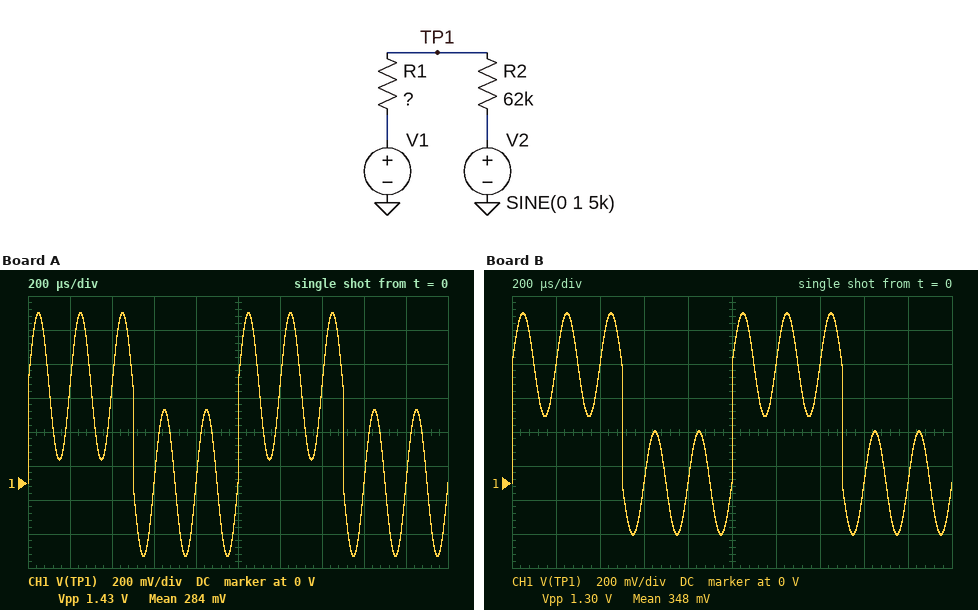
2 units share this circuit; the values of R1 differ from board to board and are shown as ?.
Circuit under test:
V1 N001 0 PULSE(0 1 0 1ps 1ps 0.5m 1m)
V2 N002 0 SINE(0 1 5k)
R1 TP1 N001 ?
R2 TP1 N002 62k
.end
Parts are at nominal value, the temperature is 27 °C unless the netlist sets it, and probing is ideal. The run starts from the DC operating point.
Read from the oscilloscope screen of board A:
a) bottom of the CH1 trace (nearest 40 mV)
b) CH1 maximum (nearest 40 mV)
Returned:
-440 mV
1.00 V
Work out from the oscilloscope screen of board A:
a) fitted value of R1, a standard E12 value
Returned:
47 kΩ
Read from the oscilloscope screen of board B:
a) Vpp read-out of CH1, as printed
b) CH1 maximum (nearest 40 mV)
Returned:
1.30 V
1.00 V
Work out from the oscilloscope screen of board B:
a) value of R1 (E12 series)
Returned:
27 kΩ
